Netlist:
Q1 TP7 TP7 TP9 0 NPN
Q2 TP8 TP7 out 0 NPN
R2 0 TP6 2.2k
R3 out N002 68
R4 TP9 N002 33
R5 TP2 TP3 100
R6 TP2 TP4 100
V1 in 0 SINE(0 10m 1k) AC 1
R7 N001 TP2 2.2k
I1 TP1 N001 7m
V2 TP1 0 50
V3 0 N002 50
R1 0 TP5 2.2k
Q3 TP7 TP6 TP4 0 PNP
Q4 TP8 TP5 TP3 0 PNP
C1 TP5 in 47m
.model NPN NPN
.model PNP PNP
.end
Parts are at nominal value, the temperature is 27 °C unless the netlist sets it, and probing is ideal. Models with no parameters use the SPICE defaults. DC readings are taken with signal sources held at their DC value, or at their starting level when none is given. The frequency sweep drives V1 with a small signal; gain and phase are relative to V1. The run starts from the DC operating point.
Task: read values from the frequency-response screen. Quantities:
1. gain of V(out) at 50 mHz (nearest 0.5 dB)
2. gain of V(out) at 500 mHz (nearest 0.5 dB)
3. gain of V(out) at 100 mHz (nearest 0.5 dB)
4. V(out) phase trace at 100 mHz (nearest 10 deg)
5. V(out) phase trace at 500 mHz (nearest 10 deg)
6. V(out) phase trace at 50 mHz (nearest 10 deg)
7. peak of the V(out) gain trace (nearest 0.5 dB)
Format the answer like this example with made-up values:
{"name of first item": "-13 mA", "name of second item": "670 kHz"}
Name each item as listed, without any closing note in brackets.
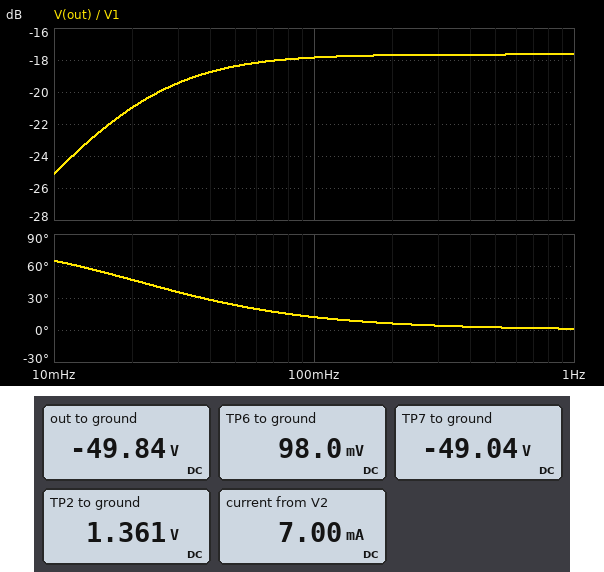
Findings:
{"gain of V(out) at 50 mHz": "-18.5 dB", "gain of V(out) at 500 mHz": "-17.5 dB", "gain of V(out) at 100 mHz": "-18.0 dB", "V(out) phase trace at 100 mHz": "10 deg", "V(out) phase trace at 500 mHz": "0 deg", "V(out) phase trace at 50 mHz": "20 deg", "peak of the V(out) gain trace": "-17.5 dB"}
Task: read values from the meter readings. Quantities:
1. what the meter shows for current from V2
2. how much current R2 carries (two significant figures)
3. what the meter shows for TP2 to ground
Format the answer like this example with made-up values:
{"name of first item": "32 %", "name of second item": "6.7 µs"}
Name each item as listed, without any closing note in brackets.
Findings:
{"what the meter shows for current from V2": "7.00 mA", "how much current R2 carries": "45 µA", "what the meter shows for TP2 to ground": "1.361 V"}
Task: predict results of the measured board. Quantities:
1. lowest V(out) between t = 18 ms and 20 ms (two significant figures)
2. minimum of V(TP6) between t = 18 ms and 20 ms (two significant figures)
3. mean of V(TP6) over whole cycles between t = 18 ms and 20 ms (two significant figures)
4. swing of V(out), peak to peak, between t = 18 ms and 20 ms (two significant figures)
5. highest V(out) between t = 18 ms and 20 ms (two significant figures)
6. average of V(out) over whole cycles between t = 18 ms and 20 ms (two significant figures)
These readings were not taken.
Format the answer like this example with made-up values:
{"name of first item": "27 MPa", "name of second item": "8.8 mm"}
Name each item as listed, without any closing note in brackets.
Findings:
{"lowest V(out) between t = 18 ms and 20 ms": "-50 V", "minimum of V(TP6) between t = 18 ms and 20 ms": "97 mV", "mean of V(TP6) over whole cycles between t = 18 ms and 20 ms": "98 mV", "swing of V(out), peak to peak, between t = 18 ms and 20 ms": "2.6 mV", "highest V(out) between t = 18 ms and 20 ms": "-50 V", "average of V(out) over whole cycles between t = 18 ms and 20 ms": "-50 V"}
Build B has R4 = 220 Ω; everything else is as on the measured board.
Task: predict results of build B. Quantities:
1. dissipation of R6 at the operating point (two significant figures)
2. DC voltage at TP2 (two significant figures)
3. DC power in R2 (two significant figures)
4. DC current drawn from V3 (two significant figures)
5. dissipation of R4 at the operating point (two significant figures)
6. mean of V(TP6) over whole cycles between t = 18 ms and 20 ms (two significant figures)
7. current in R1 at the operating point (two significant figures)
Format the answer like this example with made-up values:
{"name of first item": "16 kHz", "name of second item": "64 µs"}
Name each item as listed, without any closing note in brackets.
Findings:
{"dissipation of R6 at the operating point": "1.2 mW", "DC voltage at TP2": "1.2 V", "DC power in R2": "2.6 µW", "DC current drawn from V3": "6.9 mA", "dissipation of R4 at the operating point": "680 µW", "mean of V(TP6) over whole cycles between t = 18 ms and 20 ms": "76 mV", "current in R1 at the operating point": "35 µA"}
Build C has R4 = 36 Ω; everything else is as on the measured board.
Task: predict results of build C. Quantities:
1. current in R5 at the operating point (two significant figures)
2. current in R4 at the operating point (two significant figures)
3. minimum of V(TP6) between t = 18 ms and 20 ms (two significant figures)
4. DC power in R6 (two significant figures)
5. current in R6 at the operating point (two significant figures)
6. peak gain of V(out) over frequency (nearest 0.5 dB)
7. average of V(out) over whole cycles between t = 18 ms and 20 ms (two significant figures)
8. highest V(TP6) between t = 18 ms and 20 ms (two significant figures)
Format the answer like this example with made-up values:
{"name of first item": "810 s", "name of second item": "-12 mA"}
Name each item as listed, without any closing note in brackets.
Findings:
{"current in R5 at the operating point": "2.6 mA", "current in R4 at the operating point": "4.3 mA", "minimum of V(TP6) between t = 18 ms and 20 ms": "95 mV", "DC power in R6": "1.9 mW", "current in R6 at the operating point": "4.4 mA", "peak gain of V(out) over frequency": "-17.0 dB", "average of V(out) over whole cycles between t = 18 ms and 20 ms": "-50 V", "highest V(TP6) between t = 18 ms and 20 ms": "97 mV"}
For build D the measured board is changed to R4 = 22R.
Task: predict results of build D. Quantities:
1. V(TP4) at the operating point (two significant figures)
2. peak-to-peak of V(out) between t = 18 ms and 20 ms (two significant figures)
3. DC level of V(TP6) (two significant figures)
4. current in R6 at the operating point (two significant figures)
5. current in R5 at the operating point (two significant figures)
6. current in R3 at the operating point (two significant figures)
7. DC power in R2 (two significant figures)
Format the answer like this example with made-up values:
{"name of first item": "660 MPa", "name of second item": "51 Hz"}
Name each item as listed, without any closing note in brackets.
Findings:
{"V(TP4) at the operating point": "920 mV", "peak-to-peak of V(out) between t = 18 ms and 20 ms": "1.8 mV", "DC level of V(TP6)": "110 mV", "current in R6 at the operating point": "4.9 mA", "current in R5 at the operating point": "2.1 mA", "current in R3 at the operating point": "1.9 mA", "DC power in R2": "5.2 µW"}
